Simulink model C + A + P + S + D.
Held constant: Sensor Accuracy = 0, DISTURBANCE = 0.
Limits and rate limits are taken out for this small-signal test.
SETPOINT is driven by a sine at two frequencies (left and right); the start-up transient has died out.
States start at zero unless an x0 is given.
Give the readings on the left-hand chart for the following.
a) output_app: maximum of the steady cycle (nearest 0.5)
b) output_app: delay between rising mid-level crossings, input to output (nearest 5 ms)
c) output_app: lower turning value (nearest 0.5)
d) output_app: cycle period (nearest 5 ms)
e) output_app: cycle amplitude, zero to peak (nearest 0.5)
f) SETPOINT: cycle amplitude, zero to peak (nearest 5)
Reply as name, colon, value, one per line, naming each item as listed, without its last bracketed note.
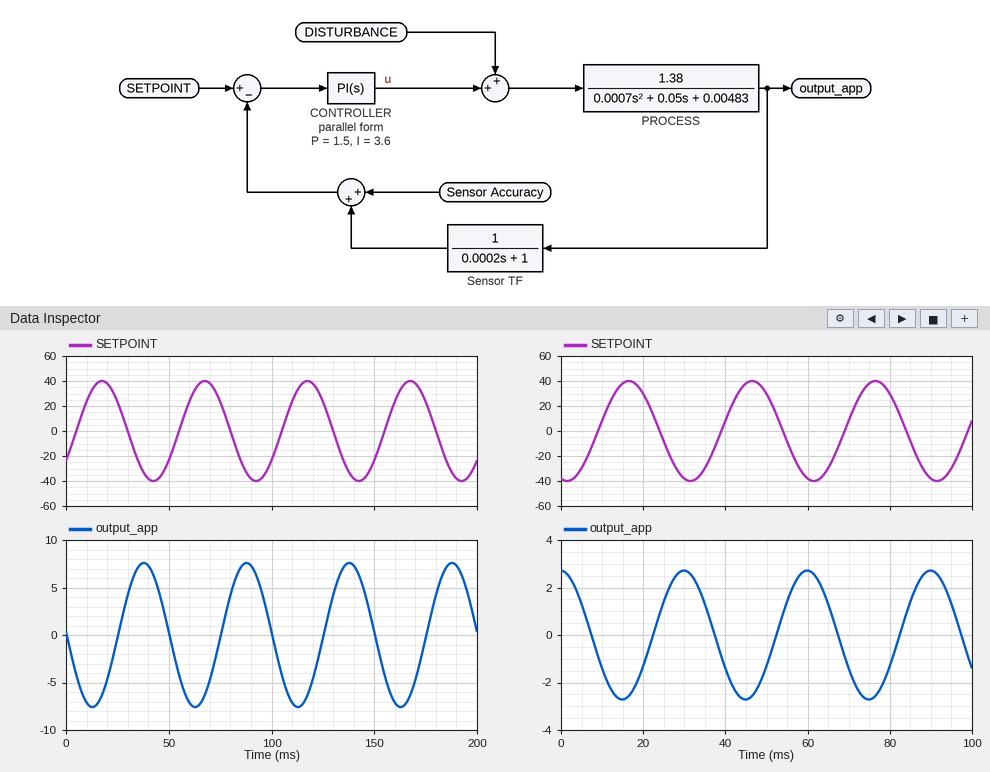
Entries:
output_app: maximum of the steady cycle: 7.5
output_app: delay between rising mid-level crossings, input to output: 20 ms
output_app: lower turning value: -7.5
output_app: cycle period: 50 ms
output_app: cycle amplitude, zero to peak: 7.5
SETPOINT: cycle amplitude, zero to peak: 40
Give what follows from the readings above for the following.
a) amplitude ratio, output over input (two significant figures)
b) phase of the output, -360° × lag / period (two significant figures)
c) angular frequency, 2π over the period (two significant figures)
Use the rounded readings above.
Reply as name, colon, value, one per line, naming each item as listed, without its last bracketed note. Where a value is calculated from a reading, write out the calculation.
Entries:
amplitude ratio, output over input: 7.5 / 40 = 0.19
phase of the output, -360° × lag / period: -360 × 20 / 50 = -140°
angular frequency, 2π over the period: 2π / 50 = 0.13 rad/ms
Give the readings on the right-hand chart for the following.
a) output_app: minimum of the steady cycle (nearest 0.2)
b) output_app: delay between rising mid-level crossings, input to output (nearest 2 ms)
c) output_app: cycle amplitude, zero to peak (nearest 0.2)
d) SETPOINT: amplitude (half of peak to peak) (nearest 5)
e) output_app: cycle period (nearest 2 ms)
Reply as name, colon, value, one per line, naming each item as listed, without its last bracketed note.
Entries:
output_app: minimum of the steady cycle: -2.8
output_app: delay between rising mid-level crossings, input to output: 14 ms
output_app: cycle amplitude, zero to peak: 2.8
SETPOINT: amplitude (half of peak to peak): 40
output_app: cycle period: 30 ms
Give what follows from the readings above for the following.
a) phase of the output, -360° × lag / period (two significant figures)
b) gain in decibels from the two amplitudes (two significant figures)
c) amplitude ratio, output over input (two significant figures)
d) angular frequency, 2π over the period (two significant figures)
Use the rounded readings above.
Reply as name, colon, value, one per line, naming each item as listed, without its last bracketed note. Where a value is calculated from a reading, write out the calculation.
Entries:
phase of the output, -360° × lag / period: -360 × 14 / 30 = -170°
gain in decibels from the two amplitudes: 20 log10(2.8 / 40) = -23 dB
amplitude ratio, output over input: 2.8 / 40 = 0.070
angular frequency, 2π over the period: 2π / 30 = 0.21 rad/ms
